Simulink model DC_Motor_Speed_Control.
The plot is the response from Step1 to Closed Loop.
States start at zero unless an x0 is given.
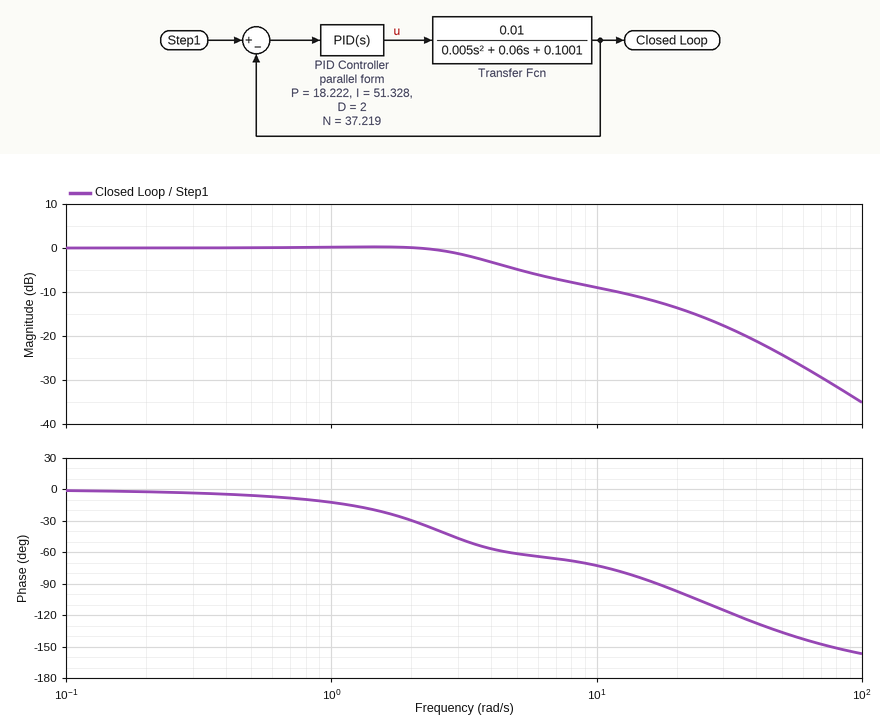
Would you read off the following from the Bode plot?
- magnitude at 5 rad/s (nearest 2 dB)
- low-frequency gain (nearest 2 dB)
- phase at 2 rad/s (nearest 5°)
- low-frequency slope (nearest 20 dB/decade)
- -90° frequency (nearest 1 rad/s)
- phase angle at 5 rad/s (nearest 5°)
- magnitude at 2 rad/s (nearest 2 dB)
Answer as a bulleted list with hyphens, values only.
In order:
- -4 dB
- 0 dB
- -30°
- 0 dB/decade
- 17 rad/s
- -60°
- 0 dB
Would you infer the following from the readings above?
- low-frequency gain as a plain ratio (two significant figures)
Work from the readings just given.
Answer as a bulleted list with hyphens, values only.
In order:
- 1.0
